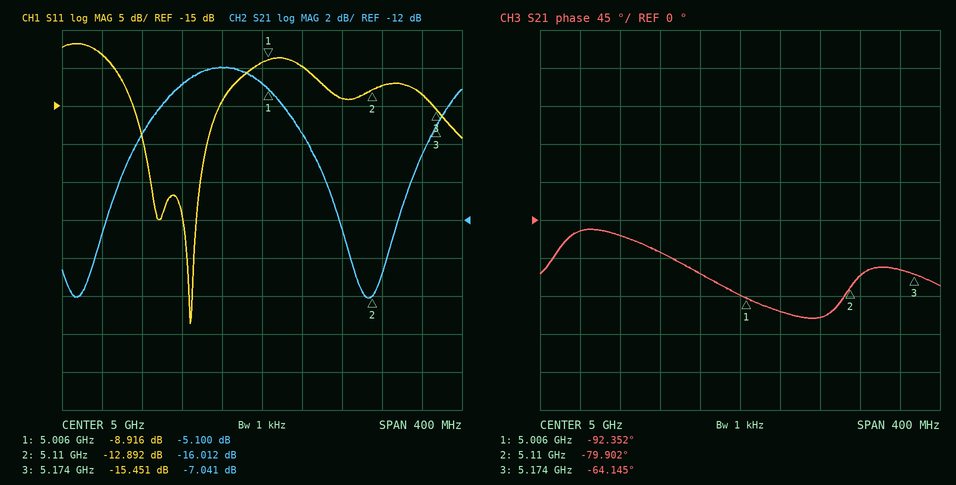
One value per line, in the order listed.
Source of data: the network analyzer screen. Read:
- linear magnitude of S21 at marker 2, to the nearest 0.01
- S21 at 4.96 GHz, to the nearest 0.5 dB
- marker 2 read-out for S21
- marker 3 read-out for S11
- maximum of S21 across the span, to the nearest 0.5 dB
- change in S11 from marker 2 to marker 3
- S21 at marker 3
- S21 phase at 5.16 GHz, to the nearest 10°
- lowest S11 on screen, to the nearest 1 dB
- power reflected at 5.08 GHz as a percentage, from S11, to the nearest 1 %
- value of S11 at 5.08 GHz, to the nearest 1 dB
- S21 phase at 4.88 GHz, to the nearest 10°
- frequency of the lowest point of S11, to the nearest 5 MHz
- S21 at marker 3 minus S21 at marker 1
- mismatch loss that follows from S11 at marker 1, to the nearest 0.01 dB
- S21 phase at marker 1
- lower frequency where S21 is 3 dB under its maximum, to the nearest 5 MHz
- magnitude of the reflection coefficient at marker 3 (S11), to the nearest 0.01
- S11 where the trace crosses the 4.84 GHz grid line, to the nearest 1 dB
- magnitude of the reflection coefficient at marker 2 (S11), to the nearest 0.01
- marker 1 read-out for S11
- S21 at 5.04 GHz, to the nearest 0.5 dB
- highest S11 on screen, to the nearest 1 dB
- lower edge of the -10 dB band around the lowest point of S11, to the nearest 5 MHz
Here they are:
0.16
-4.0 dB
-16.012 dB
-15.451 dB
-4.0 dB
-2.559 dB
-7.041 dB
-60°
-44 dB
4 %
-14 dB
-20°
4.930 GHz
-1.941 dB
0.60 dB
-92.352°
4.885 GHz
0.17
-8 dB
0.23
-8.916 dB
-7.5 dB
-7 dB
4.850 GHz
